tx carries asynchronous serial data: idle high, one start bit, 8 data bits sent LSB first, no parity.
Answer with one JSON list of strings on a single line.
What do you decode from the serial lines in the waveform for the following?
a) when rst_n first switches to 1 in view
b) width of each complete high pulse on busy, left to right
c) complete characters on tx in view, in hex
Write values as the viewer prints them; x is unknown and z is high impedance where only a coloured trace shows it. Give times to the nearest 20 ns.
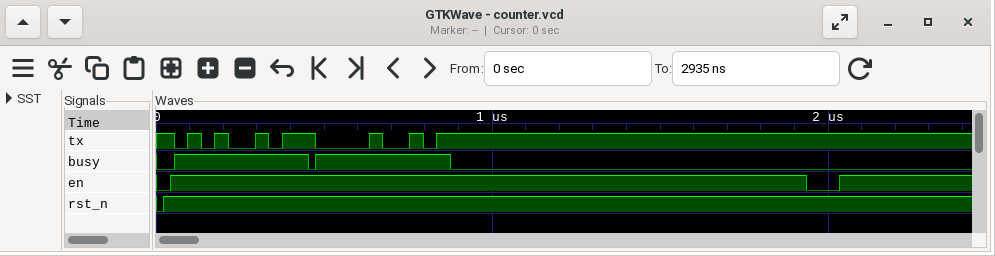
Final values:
["20 ns", "400 ns, 400 ns", "A5, 48"]
